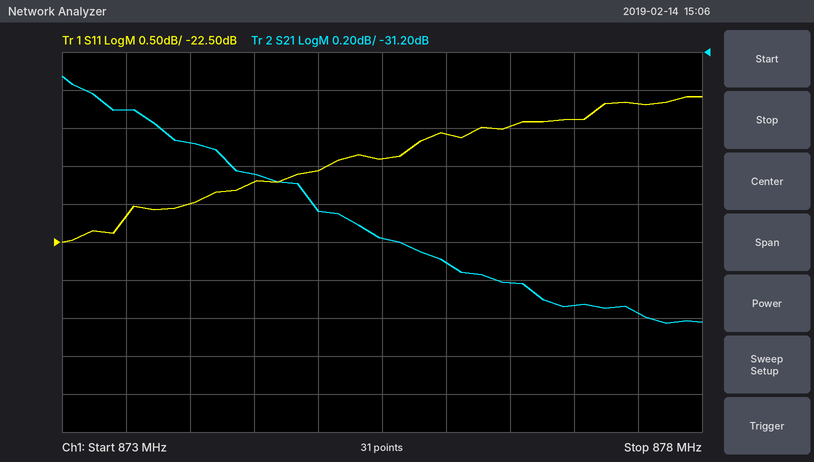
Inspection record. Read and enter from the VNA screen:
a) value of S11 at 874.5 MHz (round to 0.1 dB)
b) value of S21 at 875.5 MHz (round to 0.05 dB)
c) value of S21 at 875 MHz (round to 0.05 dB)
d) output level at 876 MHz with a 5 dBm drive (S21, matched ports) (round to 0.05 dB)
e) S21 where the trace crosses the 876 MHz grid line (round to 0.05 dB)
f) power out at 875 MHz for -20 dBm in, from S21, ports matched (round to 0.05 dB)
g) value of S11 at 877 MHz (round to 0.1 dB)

-21.7 dB
-32.20 dB
-32.05 dB
-27.30 dBm
-32.30 dB
-52.05 dBm
-20.9 dB
